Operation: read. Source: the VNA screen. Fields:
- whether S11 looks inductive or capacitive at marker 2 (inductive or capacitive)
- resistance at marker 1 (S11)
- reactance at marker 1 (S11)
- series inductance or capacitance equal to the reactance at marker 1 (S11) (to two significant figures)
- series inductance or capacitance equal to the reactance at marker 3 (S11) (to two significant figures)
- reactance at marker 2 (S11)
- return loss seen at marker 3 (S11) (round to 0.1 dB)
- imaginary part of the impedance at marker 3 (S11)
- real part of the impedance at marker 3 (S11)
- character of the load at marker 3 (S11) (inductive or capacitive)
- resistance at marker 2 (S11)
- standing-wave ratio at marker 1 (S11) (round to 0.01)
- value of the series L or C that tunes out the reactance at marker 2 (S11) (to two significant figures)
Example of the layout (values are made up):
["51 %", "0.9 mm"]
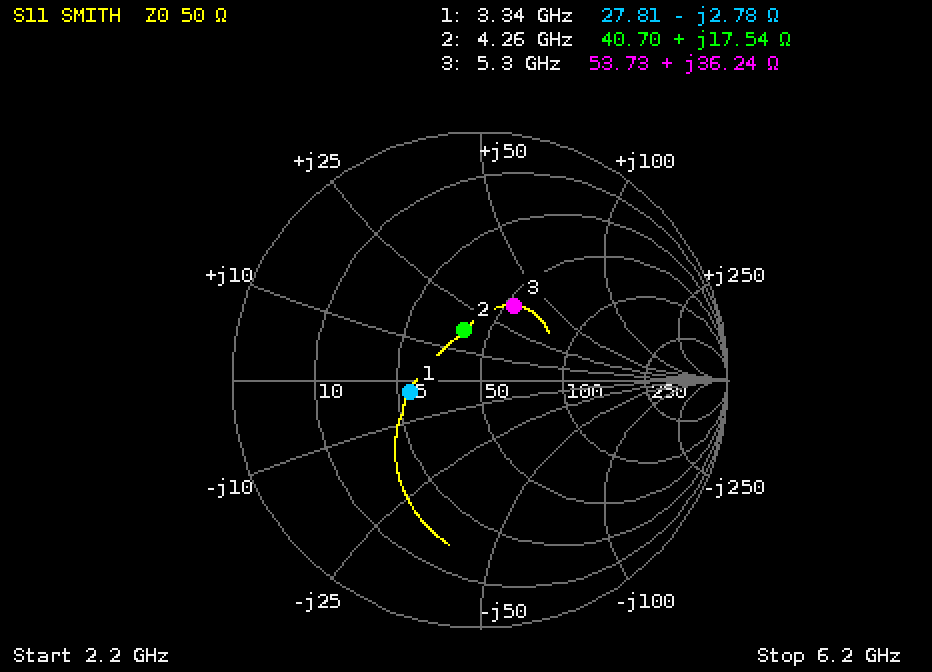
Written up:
["inductive", "27.81 Ω", "-2.78 Ω", "17 pF", "1.1 nH", "+17.54 Ω", "9.6 dB", "+36.24 Ω", "53.73 Ω", "inductive", "40.70 Ω", "1.81", "2.1 pF"]
